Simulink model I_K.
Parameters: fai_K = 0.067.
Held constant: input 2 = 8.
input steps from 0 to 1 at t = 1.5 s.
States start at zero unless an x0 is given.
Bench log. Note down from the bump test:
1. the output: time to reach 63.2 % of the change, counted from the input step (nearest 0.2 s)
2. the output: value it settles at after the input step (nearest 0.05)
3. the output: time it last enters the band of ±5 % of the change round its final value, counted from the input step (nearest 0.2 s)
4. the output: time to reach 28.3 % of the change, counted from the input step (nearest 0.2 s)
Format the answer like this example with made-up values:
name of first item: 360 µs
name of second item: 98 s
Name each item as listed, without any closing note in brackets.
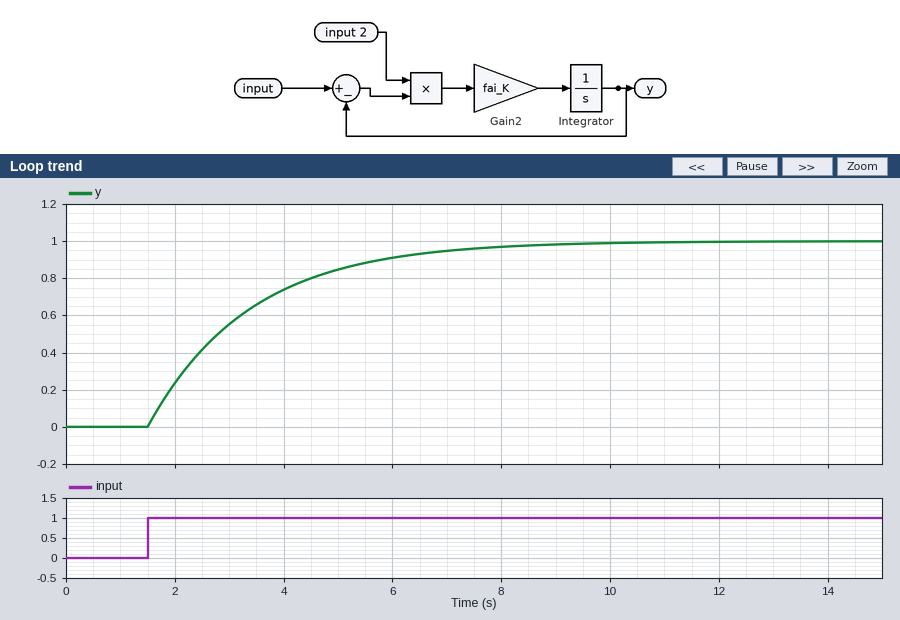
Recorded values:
the output: time to reach 63.2 % of the change, counted from the input step: 1.8 s
the output: value it settles at after the input step: 1.00
the output: time it last enters the band of ±5 % of the change round its final value, counted from the input step: 5.6 s
the output: time to reach 28.3 % of the change, counted from the input step: 0.6 s
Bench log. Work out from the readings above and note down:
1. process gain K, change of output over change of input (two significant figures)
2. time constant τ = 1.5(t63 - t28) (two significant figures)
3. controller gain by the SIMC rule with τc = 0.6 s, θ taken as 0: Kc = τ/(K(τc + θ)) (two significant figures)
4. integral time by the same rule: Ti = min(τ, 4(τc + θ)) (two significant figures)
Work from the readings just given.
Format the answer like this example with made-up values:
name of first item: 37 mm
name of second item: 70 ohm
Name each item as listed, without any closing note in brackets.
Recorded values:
process gain K, change of output over change of input: 1.0
time constant τ = 1.5(t63 - t28): 1.8 s
controller gain by the SIMC rule with τc = 0.6 s, θ taken as 0: Kc = τ/(K(τc + θ)): 3.0
integral time by the same rule: Ti = min(τ, 4(τc + θ)): 1.8 s
